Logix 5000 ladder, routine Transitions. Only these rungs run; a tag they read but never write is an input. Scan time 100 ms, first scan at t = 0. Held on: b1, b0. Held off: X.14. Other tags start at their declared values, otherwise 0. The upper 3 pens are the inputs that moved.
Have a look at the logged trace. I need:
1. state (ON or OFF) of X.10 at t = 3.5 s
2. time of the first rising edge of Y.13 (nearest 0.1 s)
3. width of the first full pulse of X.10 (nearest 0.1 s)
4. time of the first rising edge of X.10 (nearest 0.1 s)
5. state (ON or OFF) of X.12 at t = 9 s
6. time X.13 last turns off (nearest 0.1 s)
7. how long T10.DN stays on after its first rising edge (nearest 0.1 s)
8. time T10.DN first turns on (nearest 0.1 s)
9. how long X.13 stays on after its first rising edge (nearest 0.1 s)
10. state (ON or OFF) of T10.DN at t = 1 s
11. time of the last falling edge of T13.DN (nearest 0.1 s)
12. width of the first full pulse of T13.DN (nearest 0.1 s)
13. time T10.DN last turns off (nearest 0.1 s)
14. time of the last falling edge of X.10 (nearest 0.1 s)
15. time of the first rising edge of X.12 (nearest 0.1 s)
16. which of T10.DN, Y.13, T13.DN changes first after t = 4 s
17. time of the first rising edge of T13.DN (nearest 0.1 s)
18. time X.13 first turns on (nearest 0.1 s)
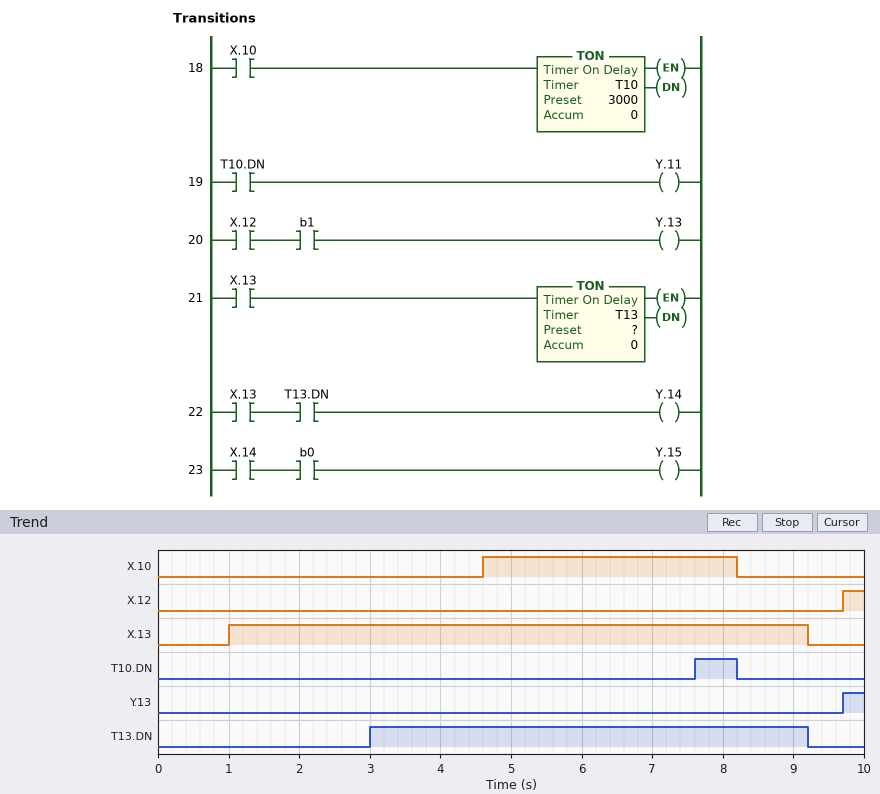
OFF
9.7 s
3.6 s
4.6 s
OFF
9.2 s
0.6 s
7.6 s
8.2 s
OFF
9.2 s
6.2 s
8.2 s
8.2 s
9.7 s
T10.DN
3.0 s
1.0 s
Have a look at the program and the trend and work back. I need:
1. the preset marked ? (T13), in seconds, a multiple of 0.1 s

2.0 s
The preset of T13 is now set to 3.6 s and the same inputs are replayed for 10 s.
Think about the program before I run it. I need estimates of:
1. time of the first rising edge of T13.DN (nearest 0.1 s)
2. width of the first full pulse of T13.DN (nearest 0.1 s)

4.6 s
4.6 s
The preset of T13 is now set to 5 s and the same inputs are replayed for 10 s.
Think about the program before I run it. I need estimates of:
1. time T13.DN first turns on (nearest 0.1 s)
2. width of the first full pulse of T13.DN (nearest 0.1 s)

6.0 s
3.2 s
